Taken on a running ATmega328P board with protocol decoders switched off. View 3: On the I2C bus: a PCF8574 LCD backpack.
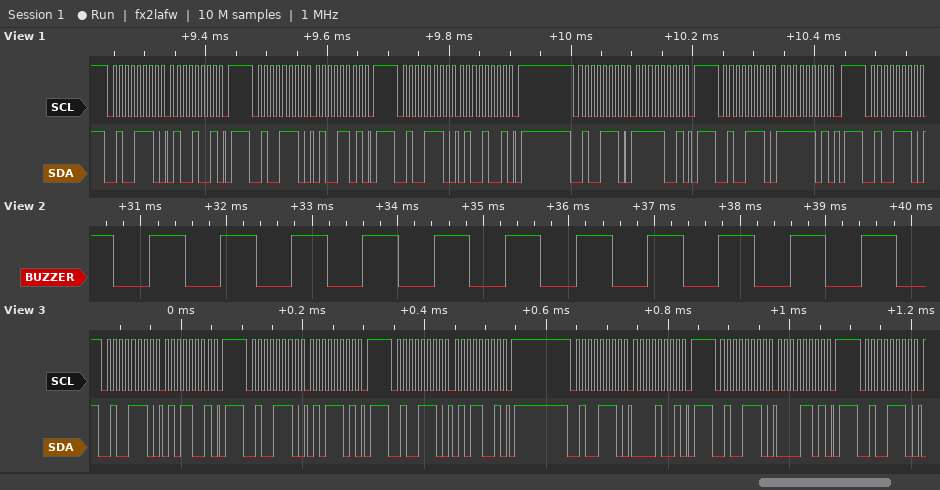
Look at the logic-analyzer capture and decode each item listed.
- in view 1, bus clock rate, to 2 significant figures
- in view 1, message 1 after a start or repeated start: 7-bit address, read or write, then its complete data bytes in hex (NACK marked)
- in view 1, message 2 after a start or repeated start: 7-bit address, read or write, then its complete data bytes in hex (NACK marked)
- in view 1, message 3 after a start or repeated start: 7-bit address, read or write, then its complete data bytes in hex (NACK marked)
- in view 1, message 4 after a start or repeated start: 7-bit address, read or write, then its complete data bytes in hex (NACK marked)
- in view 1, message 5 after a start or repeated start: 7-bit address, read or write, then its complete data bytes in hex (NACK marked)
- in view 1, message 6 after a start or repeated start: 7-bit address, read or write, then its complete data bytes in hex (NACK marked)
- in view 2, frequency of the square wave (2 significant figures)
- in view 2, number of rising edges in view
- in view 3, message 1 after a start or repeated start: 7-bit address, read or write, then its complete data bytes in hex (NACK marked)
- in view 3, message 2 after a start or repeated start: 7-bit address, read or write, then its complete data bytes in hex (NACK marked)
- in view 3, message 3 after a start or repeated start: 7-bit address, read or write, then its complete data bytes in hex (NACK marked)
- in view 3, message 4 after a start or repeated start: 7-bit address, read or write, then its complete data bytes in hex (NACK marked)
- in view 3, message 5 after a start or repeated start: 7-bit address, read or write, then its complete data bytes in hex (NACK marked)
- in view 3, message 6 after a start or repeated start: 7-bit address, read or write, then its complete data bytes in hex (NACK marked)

100 kHz
0x27 write: 49
0x27 write: 4D
0x27 write: 49
0x27 write: F9
0x27 write: FD
0x27 write
1.2 kHz
11
0x27 write: 59
0x27 write: 5D
0x27 write: 59
0x27 write: 09
0x27 write: 0D
0x27 write
